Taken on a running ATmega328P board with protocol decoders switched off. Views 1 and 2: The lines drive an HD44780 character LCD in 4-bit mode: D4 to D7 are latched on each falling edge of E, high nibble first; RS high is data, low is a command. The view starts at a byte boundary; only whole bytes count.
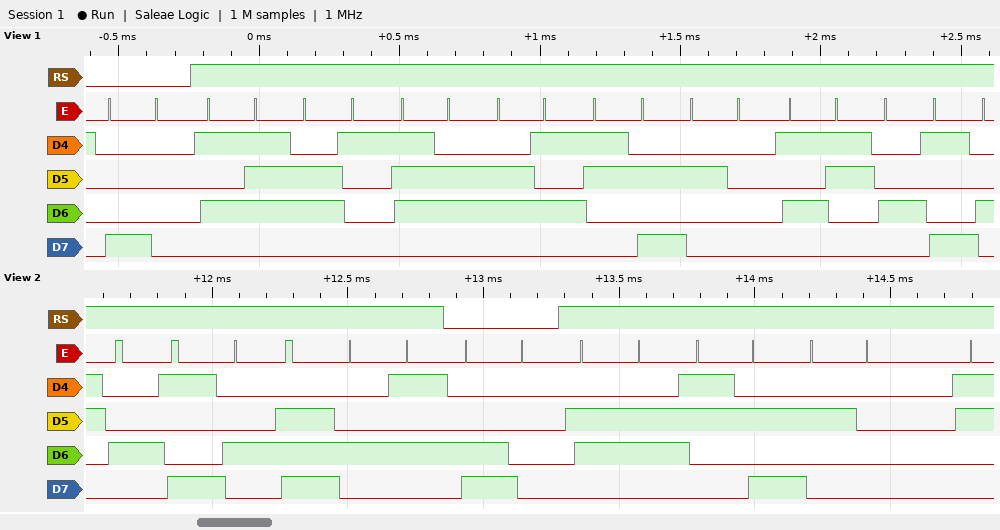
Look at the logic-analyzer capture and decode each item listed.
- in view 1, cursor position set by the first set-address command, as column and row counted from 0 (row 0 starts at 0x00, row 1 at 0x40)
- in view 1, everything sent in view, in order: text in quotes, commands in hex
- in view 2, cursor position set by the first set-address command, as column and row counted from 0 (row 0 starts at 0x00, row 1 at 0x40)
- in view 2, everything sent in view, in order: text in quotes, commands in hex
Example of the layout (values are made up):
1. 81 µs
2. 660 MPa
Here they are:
1. column 0, row 0
2. 0x80 "Wave: SI"
3. column 0, row 1
4. "INE" 0xC0 "f: "
